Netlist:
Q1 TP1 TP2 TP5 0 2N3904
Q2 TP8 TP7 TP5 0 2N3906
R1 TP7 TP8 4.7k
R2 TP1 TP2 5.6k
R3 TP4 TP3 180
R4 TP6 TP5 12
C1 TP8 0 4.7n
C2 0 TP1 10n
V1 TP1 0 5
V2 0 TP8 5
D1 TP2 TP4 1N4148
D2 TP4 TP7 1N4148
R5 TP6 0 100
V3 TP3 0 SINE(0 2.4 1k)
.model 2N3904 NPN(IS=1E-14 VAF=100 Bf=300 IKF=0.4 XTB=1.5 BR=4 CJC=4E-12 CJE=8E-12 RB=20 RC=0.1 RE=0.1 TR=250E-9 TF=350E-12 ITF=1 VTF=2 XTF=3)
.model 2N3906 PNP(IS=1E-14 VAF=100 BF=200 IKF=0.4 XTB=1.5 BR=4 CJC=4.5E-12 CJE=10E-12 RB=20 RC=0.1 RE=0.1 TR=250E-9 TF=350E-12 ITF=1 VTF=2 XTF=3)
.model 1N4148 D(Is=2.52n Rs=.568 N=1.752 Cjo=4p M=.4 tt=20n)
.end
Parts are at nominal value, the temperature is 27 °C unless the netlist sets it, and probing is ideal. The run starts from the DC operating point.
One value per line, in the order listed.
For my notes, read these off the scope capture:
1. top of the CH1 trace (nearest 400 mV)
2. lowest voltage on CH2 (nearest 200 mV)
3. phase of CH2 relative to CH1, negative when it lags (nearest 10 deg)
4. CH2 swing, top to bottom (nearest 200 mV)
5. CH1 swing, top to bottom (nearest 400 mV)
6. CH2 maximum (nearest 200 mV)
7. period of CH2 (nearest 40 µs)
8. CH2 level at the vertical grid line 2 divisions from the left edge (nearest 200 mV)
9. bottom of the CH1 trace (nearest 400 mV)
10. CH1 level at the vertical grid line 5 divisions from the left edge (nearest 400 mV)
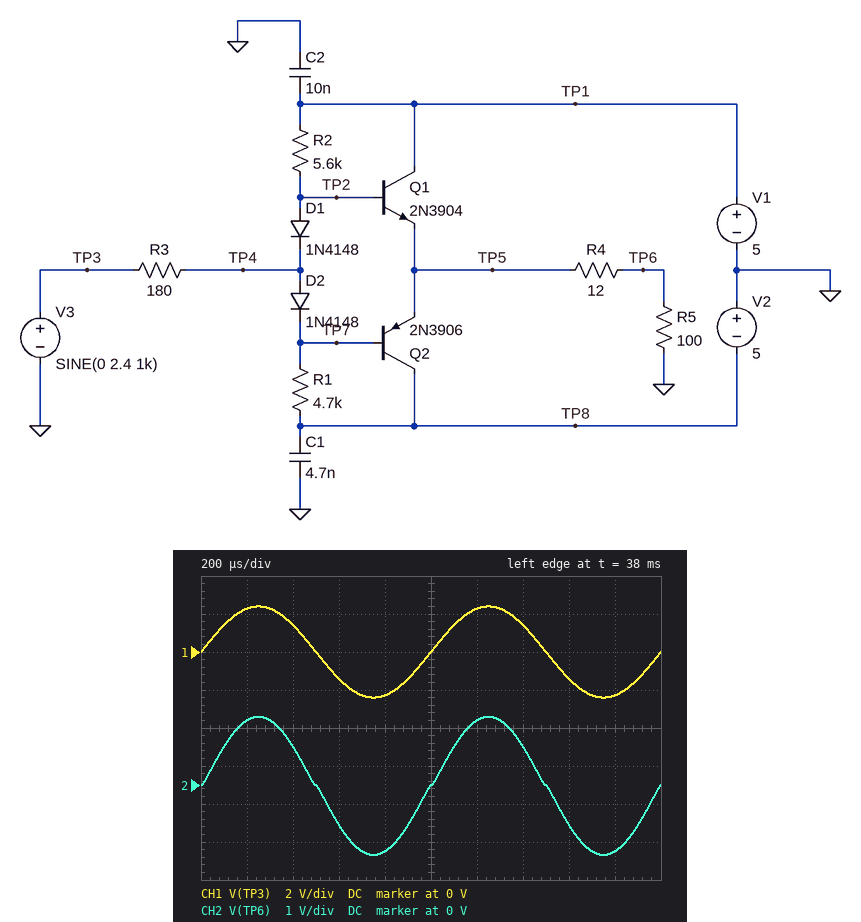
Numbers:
2.4 V
-1.8 V
0 deg
3.6 V
4.8 V
1.8 V
1.00 ms
1.0 V
-2.4 V
0 V
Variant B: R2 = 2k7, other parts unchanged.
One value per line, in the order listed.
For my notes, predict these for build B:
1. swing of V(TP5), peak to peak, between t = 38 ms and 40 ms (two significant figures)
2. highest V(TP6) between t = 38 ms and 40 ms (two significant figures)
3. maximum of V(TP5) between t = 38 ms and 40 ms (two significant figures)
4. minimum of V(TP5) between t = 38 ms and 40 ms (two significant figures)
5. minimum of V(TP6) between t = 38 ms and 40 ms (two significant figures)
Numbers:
4.0 V
1.9 V
2.1 V
-1.9 V
-1.7 V
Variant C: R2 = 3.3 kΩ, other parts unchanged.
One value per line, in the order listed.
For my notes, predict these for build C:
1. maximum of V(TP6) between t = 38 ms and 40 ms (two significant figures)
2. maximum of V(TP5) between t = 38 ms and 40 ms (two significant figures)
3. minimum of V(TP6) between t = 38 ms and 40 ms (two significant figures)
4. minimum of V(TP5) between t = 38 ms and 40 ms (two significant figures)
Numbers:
1.9 V
2.1 V
-1.7 V
-1.9 V
